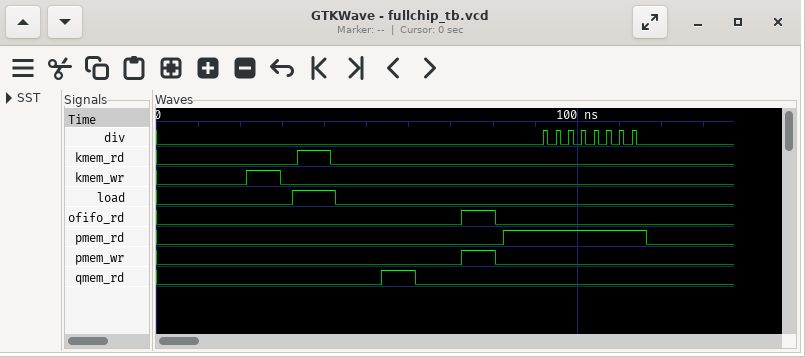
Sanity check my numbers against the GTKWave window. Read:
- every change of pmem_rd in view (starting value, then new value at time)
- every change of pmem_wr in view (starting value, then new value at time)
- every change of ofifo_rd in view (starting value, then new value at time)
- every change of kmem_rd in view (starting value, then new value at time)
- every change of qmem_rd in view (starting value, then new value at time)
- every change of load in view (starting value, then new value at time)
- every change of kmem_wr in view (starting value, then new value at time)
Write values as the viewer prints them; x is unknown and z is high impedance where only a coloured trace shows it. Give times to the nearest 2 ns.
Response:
0, 1 at 82 ns, 0 at 116 ns
0, 1 at 72 ns, 0 at 80 ns
0, 1 at 72 ns, 0 at 80 ns
0, 1 at 34 ns, 0 at 42 ns
0, 1 at 54 ns, 0 at 62 ns
0, 1 at 32 ns, 0 at 42 ns
0, 1 at 22 ns, 0 at 30 ns
